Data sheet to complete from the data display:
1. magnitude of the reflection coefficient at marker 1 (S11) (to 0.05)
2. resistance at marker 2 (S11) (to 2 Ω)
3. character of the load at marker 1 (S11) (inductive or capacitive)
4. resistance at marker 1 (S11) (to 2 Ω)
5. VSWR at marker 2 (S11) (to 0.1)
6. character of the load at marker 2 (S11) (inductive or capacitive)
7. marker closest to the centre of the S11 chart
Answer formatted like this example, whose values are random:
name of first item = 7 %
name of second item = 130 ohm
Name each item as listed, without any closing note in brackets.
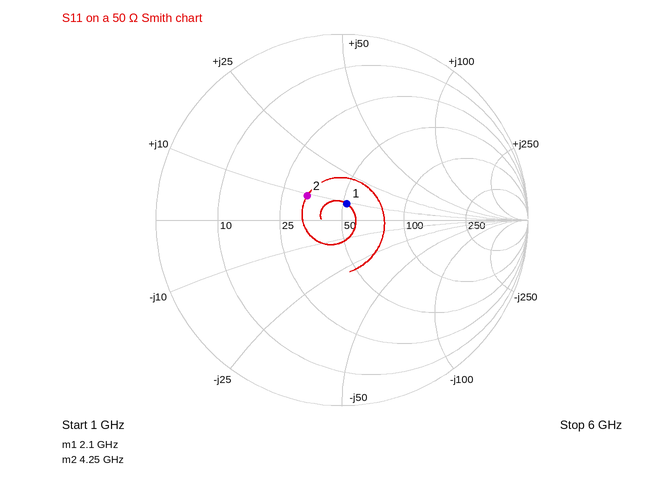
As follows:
magnitude of the reflection coefficient at marker 1 (S11) = 0.10
resistance at marker 2 (S11) = 34 Ω
character of the load at marker 1 (S11) = inductive
resistance at marker 1 (S11) = 52 Ω
VSWR at marker 2 (S11) = 1.6
character of the load at marker 2 (S11) = inductive
marker closest to the centre of the S11 chart = marker 1
